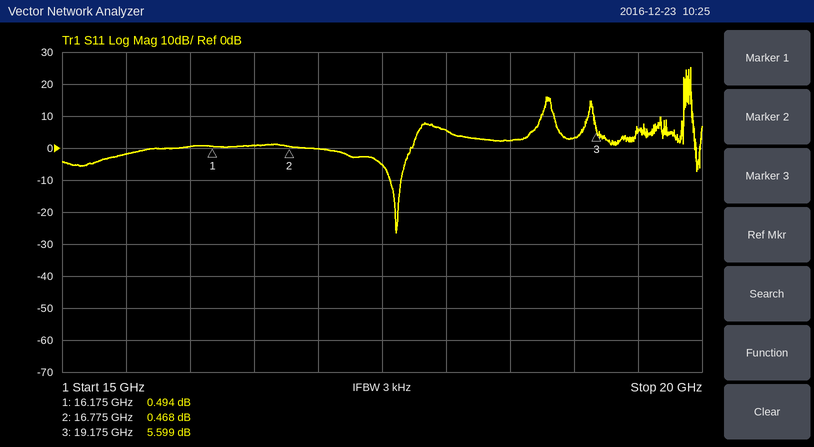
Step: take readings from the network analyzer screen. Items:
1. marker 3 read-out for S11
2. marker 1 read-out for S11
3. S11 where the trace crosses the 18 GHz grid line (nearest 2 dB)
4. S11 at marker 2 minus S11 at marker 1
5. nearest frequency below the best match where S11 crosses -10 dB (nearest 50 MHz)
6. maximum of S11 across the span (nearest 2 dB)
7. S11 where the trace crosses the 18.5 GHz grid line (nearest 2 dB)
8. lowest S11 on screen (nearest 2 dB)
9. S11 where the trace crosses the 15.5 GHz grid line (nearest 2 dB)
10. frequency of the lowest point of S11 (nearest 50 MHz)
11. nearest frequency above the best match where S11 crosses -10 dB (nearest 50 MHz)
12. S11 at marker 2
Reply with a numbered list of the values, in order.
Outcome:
1. 5.599 dB
2. 0.494 dB
3. 6 dB
4. -0.026 dB
5. 17.55 GHz
6. 26 dB
7. 2 dB
8. -26 dB
9. -2 dB
10. 17.60 GHz
11. 17.65 GHz
12. 0.468 dB
